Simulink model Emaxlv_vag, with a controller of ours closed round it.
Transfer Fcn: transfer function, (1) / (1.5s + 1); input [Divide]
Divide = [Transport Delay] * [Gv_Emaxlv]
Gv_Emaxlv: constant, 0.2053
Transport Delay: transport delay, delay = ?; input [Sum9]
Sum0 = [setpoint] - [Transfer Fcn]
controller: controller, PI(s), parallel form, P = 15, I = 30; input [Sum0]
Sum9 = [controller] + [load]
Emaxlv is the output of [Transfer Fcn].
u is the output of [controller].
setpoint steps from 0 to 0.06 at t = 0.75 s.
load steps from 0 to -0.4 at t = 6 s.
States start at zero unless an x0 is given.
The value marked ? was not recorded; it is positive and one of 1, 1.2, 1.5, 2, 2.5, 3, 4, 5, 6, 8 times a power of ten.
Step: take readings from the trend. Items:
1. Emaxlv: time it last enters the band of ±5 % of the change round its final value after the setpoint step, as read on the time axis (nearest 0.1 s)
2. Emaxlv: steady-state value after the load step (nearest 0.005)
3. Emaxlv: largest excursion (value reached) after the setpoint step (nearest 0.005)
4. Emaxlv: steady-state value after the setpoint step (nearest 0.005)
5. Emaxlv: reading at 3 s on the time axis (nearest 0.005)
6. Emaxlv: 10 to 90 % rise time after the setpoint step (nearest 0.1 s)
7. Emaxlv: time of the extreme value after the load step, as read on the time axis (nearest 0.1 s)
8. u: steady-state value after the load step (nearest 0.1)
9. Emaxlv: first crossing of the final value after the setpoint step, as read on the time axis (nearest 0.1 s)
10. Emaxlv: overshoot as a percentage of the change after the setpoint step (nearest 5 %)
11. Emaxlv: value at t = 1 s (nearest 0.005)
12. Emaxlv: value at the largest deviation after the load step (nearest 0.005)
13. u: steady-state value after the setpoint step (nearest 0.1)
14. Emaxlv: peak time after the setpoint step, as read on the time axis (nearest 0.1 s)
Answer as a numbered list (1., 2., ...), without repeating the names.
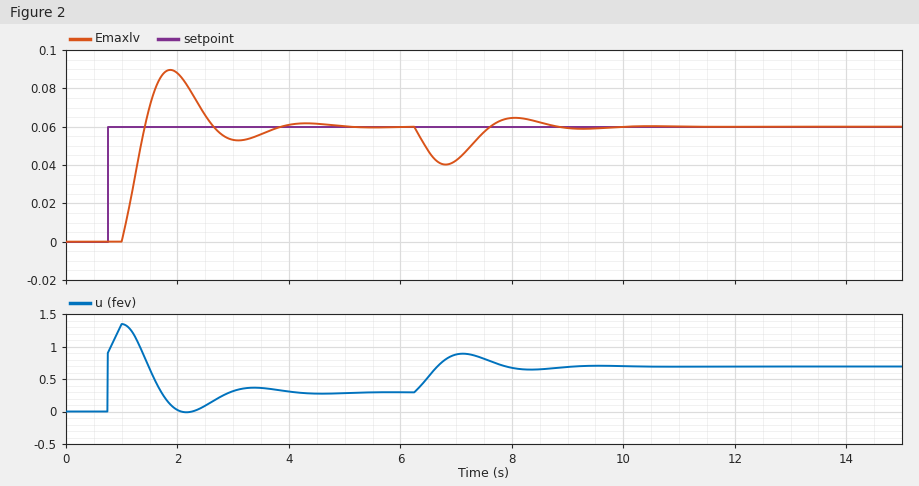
1. 3.6 s
2. 0.060
3. 0.090
4. 0.060
5. 0.055
6. 0.3 s
7. 6.8 s
8. 0.7
9. 1.4 s
10. 50 %
11. 0.000
12. 0.040
13. 0.3
14. 1.9 s
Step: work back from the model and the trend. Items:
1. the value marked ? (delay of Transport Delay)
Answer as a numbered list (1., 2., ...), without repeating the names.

1. 0.25
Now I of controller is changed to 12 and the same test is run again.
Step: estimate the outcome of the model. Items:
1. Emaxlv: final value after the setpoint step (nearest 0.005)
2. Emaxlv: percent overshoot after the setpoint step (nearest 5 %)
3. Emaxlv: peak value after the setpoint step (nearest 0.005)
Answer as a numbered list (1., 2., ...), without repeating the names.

1. 0.060
2. 10 %
3. 0.065
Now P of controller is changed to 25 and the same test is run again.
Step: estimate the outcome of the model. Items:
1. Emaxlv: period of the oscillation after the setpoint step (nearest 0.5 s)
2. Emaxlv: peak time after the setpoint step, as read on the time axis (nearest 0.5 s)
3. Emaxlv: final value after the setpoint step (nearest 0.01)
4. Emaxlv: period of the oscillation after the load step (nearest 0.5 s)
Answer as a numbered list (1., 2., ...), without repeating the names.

1. 1.5 s
2. 1.5 s
3. 0.06
4. 1.5 s
